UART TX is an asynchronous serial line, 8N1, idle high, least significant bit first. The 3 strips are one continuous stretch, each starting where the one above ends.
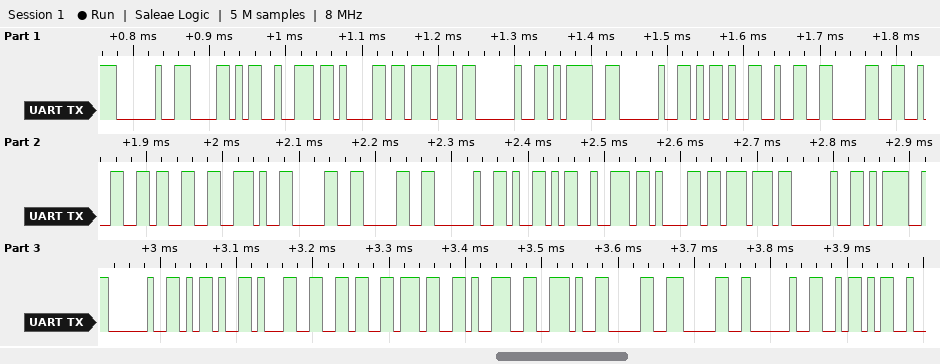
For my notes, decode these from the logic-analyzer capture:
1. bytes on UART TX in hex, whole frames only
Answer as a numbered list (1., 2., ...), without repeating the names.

1. 20 58 72 61 77 20 3D 20 2D 32 30 32 33 2E 30 30 20 59 72 61 77 20 3D 20 2D 31 36 37 39 2E 30 30 20 5A
